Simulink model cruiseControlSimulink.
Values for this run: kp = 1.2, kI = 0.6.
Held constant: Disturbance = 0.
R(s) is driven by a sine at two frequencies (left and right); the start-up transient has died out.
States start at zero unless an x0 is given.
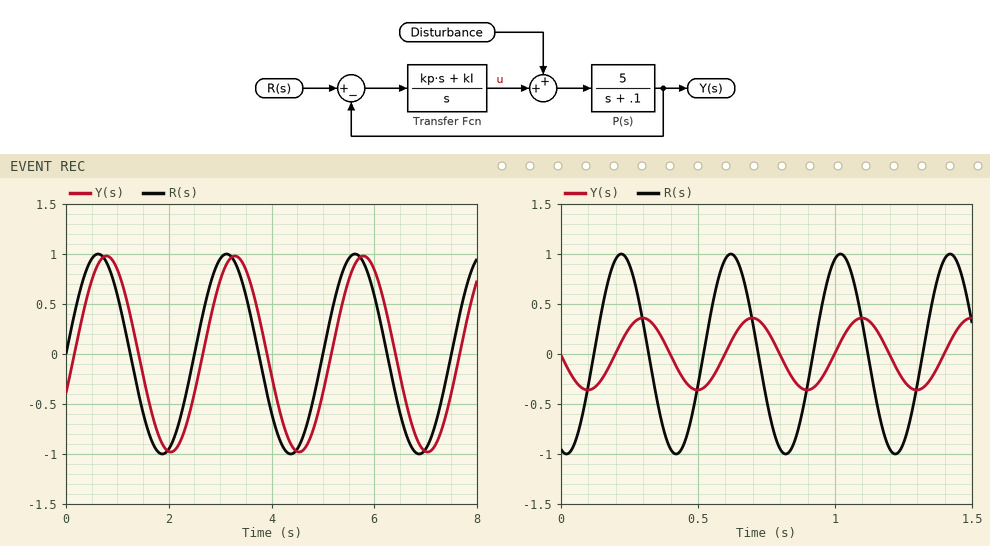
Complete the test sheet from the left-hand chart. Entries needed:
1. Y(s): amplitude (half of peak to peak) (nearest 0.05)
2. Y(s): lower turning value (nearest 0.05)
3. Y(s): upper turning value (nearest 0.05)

1.00
-1.00
1.00
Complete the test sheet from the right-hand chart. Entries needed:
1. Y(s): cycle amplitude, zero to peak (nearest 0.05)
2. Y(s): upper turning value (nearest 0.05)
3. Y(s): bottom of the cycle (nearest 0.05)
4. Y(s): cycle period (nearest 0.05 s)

0.35
0.35
-0.35
0.40 s
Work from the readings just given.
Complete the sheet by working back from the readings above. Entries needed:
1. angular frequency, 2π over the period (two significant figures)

16 rad/s
